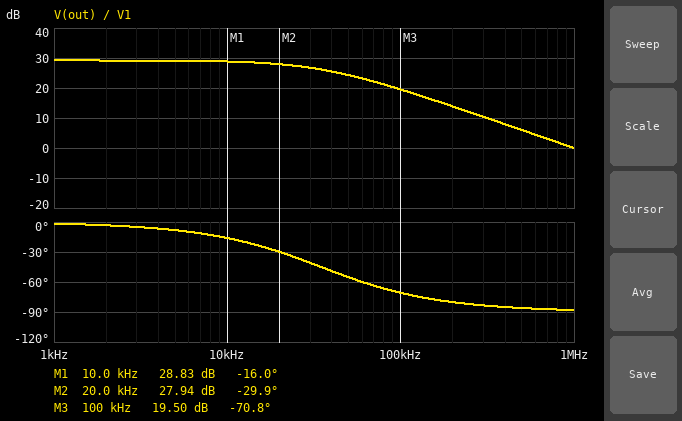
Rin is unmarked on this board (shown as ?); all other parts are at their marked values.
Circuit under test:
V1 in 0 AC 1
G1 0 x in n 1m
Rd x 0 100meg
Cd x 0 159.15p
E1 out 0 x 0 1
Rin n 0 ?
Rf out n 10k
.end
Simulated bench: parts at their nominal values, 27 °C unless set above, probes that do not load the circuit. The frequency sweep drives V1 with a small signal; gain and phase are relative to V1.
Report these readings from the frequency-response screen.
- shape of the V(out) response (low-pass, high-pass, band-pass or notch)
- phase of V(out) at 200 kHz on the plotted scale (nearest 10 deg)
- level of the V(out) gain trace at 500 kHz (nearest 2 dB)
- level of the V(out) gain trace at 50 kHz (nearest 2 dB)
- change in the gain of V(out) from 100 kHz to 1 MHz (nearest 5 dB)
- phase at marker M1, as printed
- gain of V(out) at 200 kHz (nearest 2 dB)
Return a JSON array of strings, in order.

["low-pass", "-80 deg", "6 dB", "24 dB", "-20 dB", "-16.0 deg", "14 dB"]
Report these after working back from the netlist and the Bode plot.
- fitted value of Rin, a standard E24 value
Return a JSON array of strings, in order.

["360 Ω"]
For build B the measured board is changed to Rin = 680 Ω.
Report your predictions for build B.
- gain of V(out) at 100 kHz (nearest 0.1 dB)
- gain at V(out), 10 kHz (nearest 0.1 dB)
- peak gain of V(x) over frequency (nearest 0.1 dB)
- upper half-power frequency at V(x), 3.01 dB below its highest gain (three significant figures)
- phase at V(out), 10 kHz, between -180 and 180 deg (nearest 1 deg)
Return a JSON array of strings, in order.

["18.5 dB", "23.8 dB", "23.9 dB", "63.7 kHz", "-9 deg"]
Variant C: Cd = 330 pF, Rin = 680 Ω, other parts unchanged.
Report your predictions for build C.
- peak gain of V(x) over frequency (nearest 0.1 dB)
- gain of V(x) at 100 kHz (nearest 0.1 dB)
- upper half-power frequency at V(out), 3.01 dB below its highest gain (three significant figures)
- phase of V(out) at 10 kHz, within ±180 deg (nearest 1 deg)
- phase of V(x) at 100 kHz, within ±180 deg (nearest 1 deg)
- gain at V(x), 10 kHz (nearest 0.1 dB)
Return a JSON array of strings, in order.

["23.9 dB", "13.3 dB", "30.7 kHz", "-18 deg", "-73 deg", "23.5 dB"]
